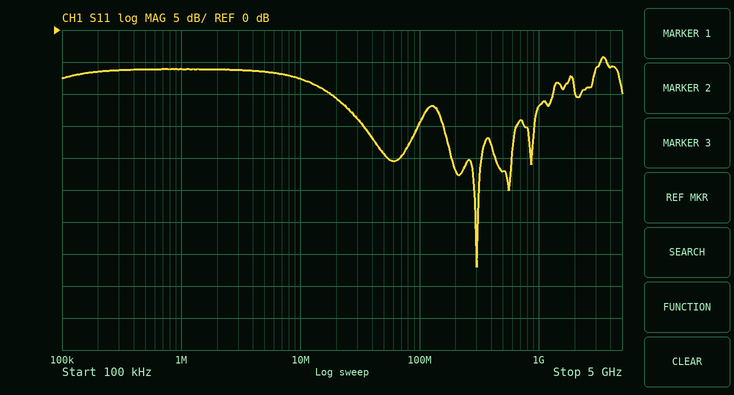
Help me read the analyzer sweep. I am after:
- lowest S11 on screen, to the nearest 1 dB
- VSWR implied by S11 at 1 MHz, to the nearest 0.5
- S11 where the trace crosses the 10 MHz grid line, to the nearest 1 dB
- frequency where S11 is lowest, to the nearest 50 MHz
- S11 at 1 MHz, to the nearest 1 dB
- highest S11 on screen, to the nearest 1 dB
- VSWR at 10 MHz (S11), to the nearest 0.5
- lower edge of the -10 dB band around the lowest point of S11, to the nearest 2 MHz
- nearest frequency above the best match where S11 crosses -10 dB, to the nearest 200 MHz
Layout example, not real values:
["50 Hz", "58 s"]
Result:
["-37 dB", "3.0", "-8 dB", "300 MHz", "-6 dB", "-4 dB", "2.5", "18 MHz", "1.4 GHz"]
